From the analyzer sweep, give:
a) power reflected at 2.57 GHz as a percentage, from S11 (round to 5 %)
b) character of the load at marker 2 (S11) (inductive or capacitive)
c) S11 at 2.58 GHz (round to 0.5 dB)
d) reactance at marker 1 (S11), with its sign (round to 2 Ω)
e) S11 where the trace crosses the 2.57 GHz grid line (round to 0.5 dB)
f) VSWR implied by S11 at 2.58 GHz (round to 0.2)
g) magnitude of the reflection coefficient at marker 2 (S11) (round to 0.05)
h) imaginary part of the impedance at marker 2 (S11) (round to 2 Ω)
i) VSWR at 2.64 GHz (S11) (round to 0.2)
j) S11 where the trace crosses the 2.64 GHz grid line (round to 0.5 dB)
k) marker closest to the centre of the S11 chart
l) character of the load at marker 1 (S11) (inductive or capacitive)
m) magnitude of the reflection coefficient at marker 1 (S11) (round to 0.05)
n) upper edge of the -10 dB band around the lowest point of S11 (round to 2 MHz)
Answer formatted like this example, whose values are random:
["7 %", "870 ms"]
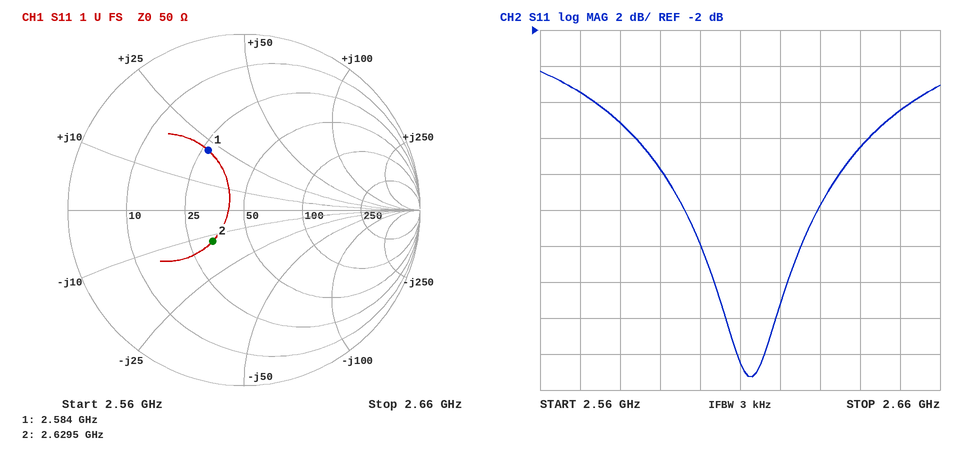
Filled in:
["30 %", "capacitive", "-7.0 dB", "+22 Ω", "-5.5 dB", "2.6", "0.25", "-12 Ω", "2.2", "-8.5 dB", "marker 2", "inductive", "0.40", "2.634 GHz"]
